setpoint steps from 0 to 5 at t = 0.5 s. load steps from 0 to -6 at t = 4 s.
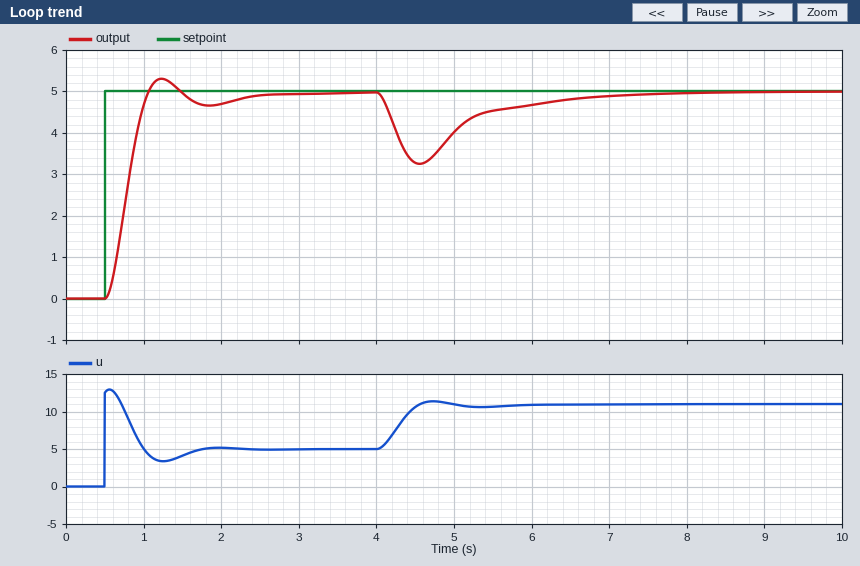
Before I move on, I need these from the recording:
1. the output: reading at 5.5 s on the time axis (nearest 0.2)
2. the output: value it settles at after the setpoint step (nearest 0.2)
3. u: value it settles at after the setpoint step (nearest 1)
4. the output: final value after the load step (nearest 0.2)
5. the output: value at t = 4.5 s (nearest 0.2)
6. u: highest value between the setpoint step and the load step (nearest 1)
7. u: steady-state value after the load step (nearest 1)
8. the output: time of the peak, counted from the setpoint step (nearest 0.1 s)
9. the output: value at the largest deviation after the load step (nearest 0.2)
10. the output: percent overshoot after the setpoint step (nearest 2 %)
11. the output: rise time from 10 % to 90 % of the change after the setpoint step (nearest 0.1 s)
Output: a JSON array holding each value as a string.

["4.6", "5.0", "5", "5.0", "3.2", "13", "11", "0.7 s", "3.2", "6 %", "0.4 s"]
